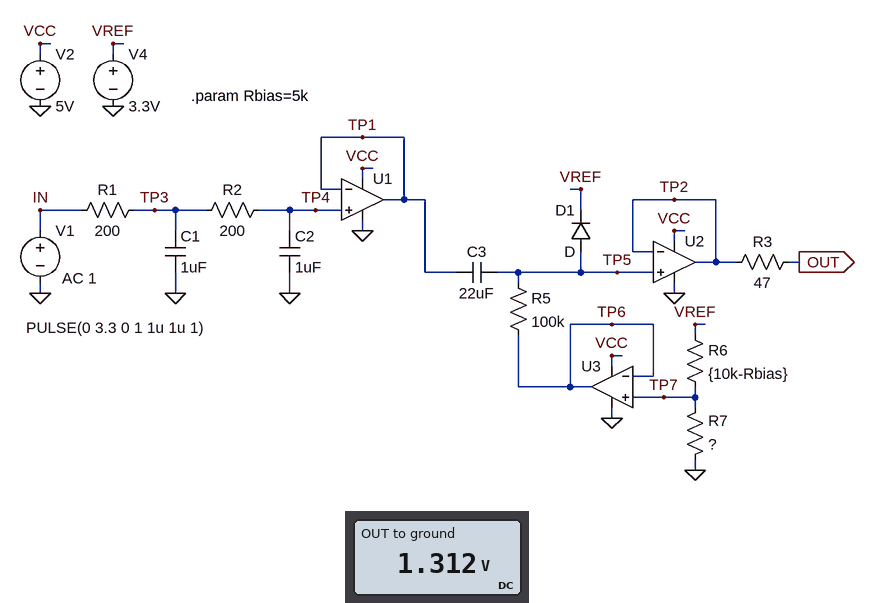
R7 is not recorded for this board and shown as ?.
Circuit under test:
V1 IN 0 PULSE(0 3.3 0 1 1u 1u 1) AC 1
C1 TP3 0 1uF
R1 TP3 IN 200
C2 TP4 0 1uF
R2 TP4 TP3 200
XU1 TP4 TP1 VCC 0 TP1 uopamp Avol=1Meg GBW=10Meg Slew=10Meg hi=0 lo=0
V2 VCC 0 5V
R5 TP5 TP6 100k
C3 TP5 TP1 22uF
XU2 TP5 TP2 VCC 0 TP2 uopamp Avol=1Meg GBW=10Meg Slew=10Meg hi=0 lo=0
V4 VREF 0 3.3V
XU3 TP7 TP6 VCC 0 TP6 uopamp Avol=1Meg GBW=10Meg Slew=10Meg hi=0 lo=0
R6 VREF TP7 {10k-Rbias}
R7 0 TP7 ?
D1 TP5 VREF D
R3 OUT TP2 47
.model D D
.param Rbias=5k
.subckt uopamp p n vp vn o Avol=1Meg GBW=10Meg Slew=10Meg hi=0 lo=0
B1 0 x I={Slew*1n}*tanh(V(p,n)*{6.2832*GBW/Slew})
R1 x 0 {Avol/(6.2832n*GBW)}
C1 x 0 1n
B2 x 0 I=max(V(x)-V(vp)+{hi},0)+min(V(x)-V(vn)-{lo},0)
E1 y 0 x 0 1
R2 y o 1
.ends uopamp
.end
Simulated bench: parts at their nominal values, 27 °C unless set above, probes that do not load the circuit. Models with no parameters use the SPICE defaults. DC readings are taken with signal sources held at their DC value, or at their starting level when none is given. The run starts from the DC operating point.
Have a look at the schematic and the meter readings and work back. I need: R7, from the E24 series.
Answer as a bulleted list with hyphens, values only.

- 3.3 kΩ
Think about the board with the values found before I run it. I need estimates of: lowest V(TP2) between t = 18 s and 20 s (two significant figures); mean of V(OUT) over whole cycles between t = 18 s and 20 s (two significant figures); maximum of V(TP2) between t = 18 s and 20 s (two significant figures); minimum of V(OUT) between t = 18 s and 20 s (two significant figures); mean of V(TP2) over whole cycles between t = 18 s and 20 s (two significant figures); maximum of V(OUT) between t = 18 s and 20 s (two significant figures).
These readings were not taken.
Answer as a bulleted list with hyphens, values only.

- -9.9 mV
- 1.3 V
- 2.8 V
- -9.9 mV
- 1.3 V
- 2.8 V
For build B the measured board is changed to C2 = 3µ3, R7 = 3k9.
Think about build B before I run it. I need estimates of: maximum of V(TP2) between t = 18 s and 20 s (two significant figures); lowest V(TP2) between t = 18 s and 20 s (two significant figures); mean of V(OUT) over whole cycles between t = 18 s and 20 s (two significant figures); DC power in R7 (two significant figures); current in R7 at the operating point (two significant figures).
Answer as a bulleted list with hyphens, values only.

- 3.0 V
- -9.4 mV
- 1.5 V
- 540 µW
- 370 µA
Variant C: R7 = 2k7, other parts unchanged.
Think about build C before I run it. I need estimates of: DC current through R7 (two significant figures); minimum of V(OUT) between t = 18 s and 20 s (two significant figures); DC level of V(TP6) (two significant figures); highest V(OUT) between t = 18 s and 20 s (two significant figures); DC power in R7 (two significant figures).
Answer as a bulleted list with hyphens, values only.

- 430 µA
- -10 mV
- 1.2 V
- 2.7 V
- 500 µW
